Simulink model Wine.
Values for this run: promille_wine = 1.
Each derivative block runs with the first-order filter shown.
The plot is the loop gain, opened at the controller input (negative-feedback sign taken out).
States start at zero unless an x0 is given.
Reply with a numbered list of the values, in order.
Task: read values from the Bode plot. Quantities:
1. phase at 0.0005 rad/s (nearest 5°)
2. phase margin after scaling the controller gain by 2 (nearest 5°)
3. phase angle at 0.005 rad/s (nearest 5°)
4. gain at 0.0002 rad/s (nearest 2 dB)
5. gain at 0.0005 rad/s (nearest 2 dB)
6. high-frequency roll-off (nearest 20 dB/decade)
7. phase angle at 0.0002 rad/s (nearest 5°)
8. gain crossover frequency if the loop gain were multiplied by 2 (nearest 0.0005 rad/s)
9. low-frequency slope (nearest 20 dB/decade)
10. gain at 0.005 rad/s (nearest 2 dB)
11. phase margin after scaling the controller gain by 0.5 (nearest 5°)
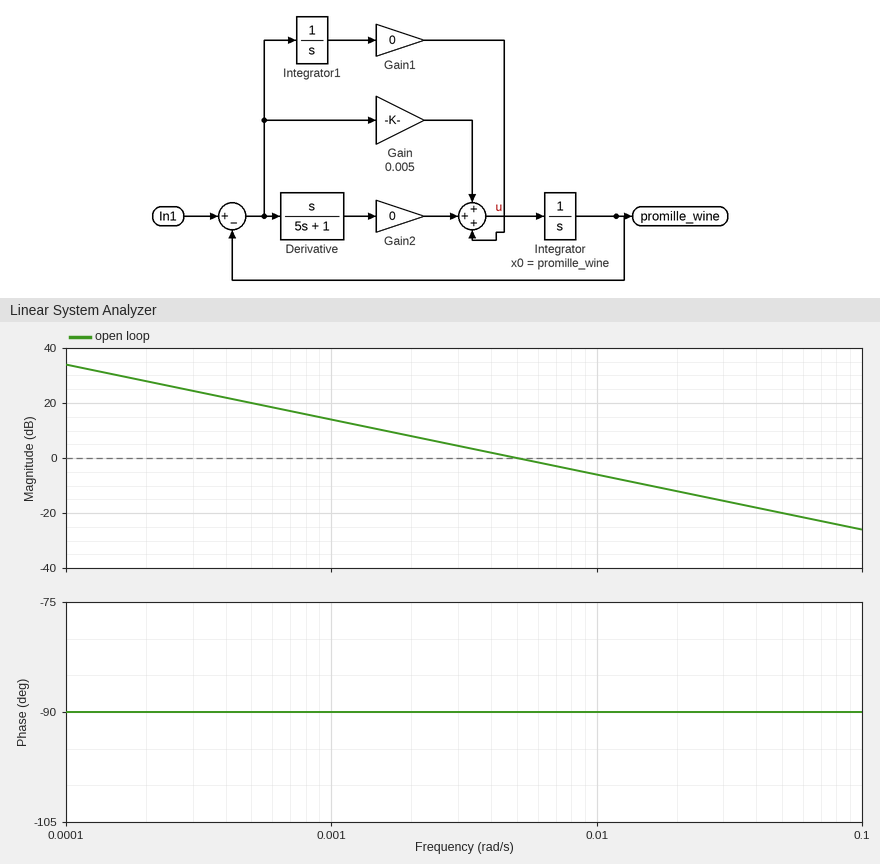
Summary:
1. -90°
2. 90°
3. -90°
4. 28 dB
5. 20 dB
6. -20 dB/decade
7. -90°
8. 0.0100 rad/s
9. -20 dB/decade
10. 0 dB
11. 90°
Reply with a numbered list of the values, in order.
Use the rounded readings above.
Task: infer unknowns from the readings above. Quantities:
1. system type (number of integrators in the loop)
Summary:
1. 1
